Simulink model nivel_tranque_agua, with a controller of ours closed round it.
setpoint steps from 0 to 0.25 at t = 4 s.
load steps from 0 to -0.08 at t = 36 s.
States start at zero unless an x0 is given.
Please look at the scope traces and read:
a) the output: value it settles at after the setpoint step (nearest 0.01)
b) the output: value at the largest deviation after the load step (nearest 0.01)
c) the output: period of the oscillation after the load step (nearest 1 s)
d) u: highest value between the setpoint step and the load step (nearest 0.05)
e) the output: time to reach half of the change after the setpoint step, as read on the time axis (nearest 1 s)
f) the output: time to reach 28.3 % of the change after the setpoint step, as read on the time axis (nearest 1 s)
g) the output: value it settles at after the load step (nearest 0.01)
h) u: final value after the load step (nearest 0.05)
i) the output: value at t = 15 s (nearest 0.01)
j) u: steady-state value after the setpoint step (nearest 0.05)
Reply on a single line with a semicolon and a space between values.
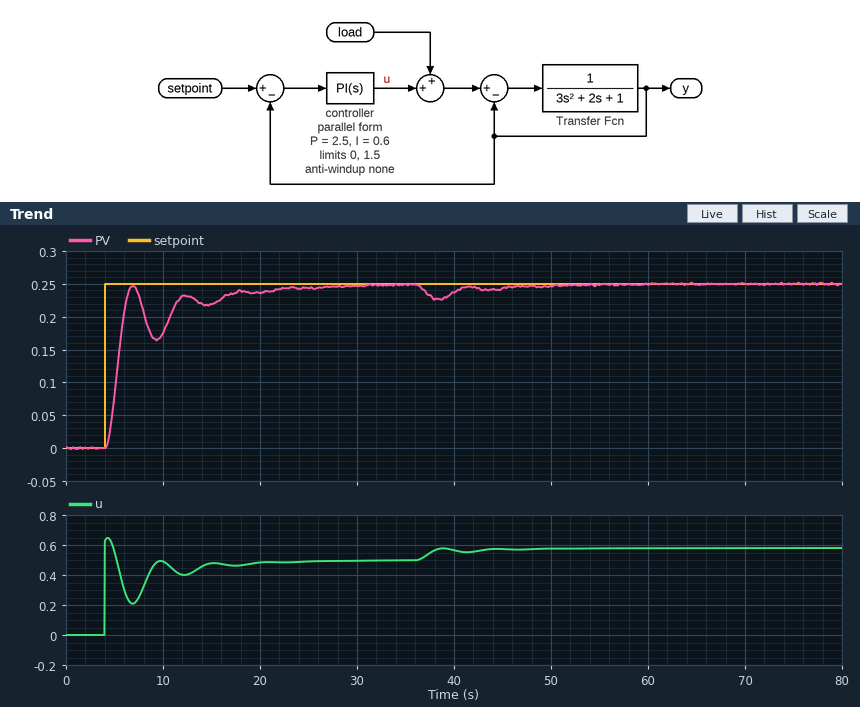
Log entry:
0.25; 0.23; 5 s; 0.65; 5 s; 5 s; 0.25; 0.60; 0.22; 0.50
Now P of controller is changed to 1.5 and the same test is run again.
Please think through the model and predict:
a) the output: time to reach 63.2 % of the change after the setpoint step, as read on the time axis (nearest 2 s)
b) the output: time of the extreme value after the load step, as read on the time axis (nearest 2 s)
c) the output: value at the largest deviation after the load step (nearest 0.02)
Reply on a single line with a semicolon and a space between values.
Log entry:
6 s; 38 s; 0.22
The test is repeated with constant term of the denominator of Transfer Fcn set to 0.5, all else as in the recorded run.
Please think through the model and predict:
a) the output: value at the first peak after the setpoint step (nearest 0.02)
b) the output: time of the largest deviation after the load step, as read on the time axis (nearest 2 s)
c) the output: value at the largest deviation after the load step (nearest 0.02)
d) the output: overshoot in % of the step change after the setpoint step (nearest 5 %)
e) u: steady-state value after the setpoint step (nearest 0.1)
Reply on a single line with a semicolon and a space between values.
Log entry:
0.28; 38 s; 0.22; 10 %; 0.4
